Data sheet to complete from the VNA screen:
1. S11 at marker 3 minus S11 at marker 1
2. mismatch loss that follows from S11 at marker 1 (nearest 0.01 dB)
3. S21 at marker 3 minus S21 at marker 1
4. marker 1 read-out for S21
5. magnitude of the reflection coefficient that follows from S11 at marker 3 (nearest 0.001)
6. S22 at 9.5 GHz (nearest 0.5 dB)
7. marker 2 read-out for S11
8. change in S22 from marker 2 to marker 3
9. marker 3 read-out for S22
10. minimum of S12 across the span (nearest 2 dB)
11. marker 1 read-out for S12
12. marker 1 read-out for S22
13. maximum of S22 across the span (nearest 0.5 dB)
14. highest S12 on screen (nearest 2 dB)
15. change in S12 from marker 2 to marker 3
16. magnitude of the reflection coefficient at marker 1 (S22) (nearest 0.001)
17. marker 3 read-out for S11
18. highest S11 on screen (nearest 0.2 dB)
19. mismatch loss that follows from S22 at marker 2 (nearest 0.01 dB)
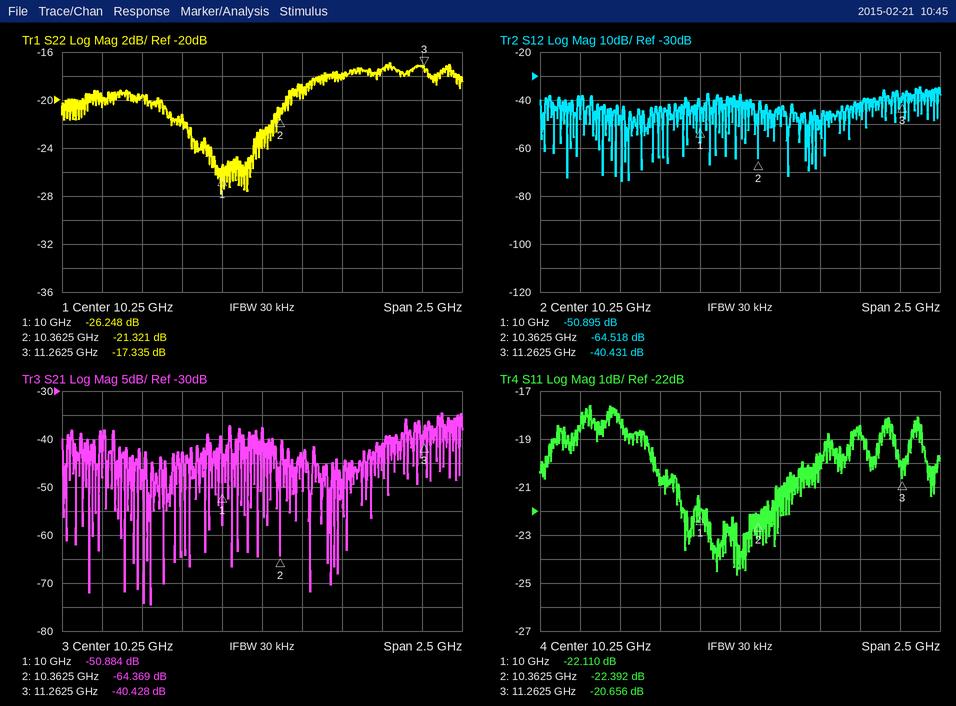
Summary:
1.454 dB
0.03 dB
10.456 dB
-50.884 dB
0.093
-19.5 dB
-22.392 dB
3.986 dB
-17.335 dB
-74 dB
-50.895 dB
-26.248 dB
-17.0 dB
-34 dB
24.087 dB
0.049
-20.656 dB
-17.6 dB
0.03 dB
